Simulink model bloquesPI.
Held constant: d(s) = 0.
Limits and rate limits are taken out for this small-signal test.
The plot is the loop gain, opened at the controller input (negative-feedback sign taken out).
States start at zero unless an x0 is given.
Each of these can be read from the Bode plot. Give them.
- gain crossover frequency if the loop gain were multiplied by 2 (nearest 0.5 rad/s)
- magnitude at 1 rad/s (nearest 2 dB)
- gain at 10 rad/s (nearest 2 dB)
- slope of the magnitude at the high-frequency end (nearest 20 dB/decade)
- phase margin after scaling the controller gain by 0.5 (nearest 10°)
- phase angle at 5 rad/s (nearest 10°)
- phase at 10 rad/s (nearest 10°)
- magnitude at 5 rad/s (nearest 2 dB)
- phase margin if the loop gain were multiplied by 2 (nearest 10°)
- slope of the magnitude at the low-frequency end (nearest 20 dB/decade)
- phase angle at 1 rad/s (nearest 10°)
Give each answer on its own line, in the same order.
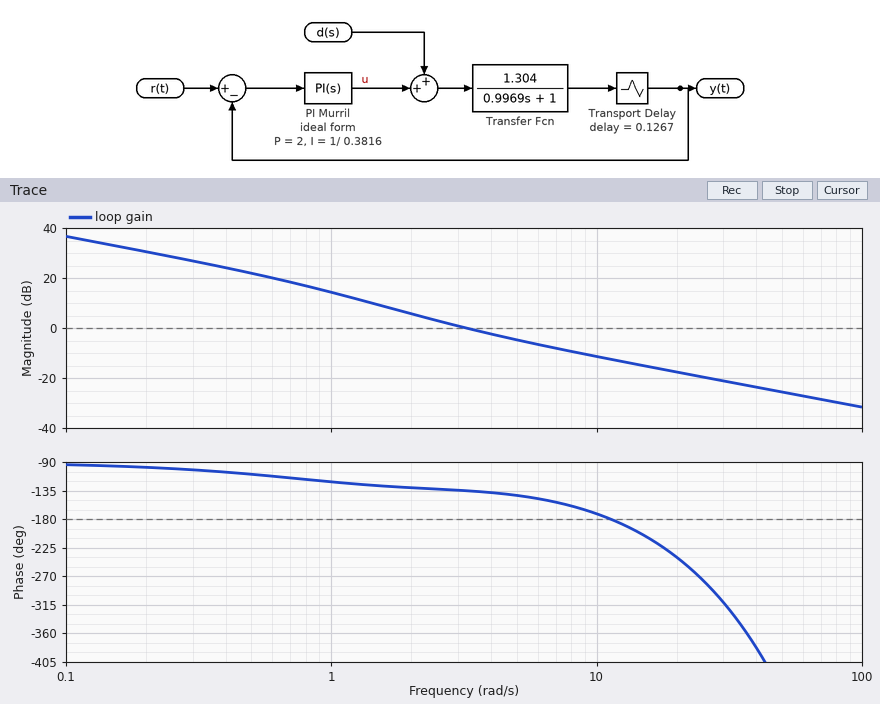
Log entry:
5.5 rad/s
14 dB
-12 dB
-20 dB/decade
50°
-140°
-170°
-4 dB
30°
-20 dB/decade
-120°
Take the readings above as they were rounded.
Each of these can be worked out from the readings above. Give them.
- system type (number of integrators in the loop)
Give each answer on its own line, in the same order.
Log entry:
1
